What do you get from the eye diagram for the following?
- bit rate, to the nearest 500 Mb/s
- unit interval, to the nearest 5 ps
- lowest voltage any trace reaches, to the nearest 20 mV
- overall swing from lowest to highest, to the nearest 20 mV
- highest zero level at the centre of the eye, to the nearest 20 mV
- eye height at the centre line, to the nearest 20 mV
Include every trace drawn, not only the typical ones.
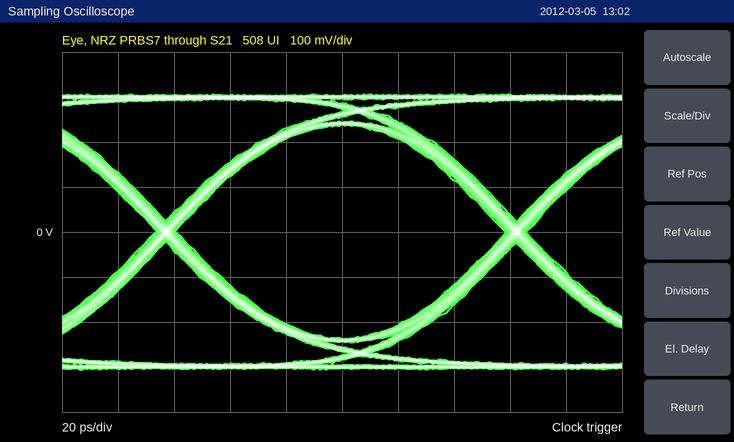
8.0 Gb/s
125 ps
-300 mV
620 mV
-240 mV
480 mV
